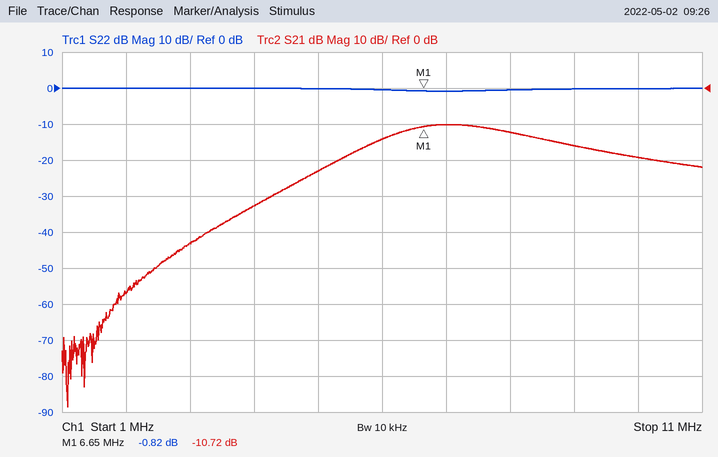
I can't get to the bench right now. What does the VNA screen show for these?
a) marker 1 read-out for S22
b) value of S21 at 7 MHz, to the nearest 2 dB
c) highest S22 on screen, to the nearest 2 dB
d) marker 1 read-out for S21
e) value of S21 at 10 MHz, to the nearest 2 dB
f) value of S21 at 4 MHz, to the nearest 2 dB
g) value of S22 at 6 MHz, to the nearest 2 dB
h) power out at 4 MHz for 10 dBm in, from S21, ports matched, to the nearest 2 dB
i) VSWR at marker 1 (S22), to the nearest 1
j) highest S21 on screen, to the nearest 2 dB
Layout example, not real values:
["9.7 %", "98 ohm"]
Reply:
["-0.82 dB", "-10 dB", "0 dB", "-10.72 dB", "-20 dB", "-32 dB", "0 dB", "-22 dBm", "21", "-10 dB"]
